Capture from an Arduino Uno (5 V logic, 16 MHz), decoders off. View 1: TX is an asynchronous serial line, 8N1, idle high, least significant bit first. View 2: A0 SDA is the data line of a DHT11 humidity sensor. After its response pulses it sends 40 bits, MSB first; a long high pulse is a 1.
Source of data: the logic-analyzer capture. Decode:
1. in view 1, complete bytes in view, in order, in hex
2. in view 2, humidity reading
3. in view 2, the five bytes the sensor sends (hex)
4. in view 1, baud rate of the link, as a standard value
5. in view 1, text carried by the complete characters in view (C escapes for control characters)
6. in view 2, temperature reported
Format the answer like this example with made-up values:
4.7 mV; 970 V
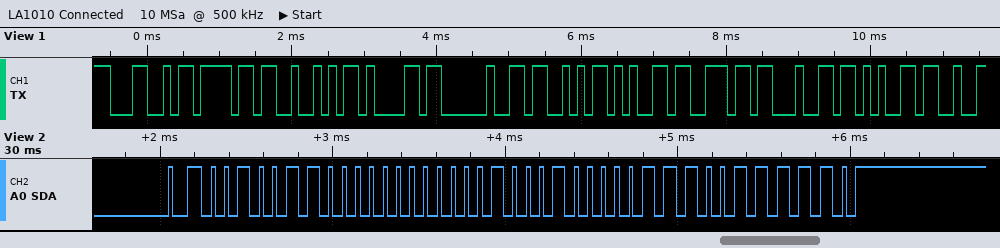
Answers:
0x4C 0x6F 0x52 0x61 0x20 0x53 0x65 0x6E 0x64 0x65; 38 %; 26 00 11 07 3E; 9600 baud; "LoRa Sende"; 17.7 °C
